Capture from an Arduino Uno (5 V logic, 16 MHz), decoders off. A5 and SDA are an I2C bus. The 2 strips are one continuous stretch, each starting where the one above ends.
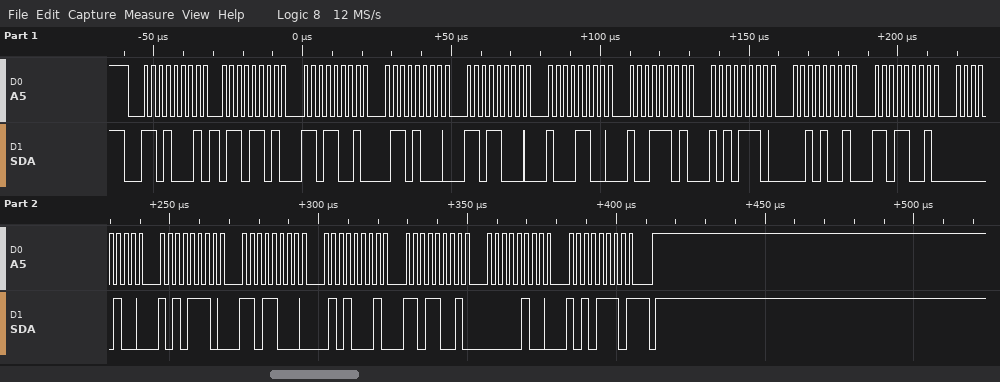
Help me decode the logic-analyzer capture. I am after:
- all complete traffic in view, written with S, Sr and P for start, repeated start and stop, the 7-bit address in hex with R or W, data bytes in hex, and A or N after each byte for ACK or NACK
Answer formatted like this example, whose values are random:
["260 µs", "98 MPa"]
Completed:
["S 68R A 6D A D9 A 68 A D8 A 8C A 9D A AE A 29 A D9 A 04 A AE A D8 A 51 A D9 A 04 A AE N P"]
